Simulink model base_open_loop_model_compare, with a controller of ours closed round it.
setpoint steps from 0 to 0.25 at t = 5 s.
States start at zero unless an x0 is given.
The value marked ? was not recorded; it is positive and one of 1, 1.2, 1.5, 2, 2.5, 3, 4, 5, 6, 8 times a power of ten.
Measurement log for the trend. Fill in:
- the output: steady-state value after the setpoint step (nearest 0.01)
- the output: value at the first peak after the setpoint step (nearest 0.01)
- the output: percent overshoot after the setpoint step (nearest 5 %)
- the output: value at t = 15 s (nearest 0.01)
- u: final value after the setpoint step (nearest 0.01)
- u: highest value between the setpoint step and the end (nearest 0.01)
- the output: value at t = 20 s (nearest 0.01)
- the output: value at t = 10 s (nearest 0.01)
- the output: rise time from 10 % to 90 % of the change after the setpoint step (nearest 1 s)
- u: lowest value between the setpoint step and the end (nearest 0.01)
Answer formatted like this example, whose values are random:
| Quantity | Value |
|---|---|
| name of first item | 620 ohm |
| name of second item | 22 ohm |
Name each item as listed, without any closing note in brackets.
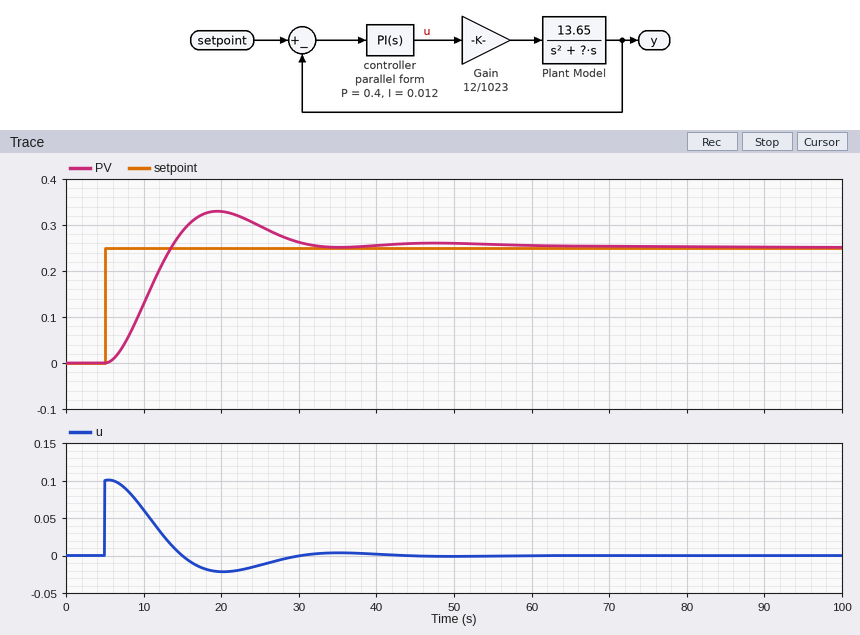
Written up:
| Quantity | Value |
|---|---|
| the output: steady-state value after the setpoint step | 0.25 |
| the output: value at the first peak after the setpoint step | 0.33 |
| the output: percent overshoot after the setpoint step | 30 % |
| the output: value at t = 15 s | 0.29 |
| u: final value after the setpoint step | 0.00 |
| u: highest value between the setpoint step and the end | 0.10 |
| the output: value at t = 20 s | 0.33 |
| the output: value at t = 10 s | 0.13 |
| the output: rise time from 10 % to 90 % of the change after the setpoint step | 6 s |
| u: lowest value between the setpoint step and the end | -0.02 |
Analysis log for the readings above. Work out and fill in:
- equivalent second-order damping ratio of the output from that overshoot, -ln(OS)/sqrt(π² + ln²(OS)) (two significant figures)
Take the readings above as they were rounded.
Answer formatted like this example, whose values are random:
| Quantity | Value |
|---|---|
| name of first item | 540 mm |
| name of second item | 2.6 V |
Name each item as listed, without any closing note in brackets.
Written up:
| Quantity | Value |
|---|---|
| equivalent second-order damping ratio of the output from that overshoot, -ln(OS)/sqrt(π² + ln²(OS)) | 0.36 |
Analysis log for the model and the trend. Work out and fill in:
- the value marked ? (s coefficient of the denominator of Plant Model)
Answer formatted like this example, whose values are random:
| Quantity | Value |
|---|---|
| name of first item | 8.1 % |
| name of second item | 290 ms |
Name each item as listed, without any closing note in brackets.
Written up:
| Quantity | Value |
|---|---|
| the value marked ? | 0.25 |
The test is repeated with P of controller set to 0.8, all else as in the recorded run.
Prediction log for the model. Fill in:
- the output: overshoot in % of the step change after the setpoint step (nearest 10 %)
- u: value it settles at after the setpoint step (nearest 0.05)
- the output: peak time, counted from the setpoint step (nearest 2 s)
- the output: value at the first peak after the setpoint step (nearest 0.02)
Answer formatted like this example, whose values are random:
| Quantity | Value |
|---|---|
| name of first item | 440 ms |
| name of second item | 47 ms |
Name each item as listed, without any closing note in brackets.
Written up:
| Quantity | Value |
|---|---|
| the output: overshoot in % of the step change after the setpoint step | 40 % |
| u: value it settles at after the setpoint step | 0.00 |
| the output: peak time, counted from the setpoint step | 10 s |
| the output: value at the first peak after the setpoint step | 0.34 |
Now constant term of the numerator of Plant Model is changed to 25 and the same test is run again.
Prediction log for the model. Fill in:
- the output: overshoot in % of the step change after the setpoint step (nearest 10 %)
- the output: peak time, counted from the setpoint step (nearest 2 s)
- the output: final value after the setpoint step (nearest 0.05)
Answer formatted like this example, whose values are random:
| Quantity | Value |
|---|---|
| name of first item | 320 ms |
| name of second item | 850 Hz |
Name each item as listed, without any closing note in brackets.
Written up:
| Quantity | Value |
|---|---|
| the output: overshoot in % of the step change after the setpoint step | 40 % |
| the output: peak time, counted from the setpoint step | 10 s |
| the output: final value after the setpoint step | 0.25 |
